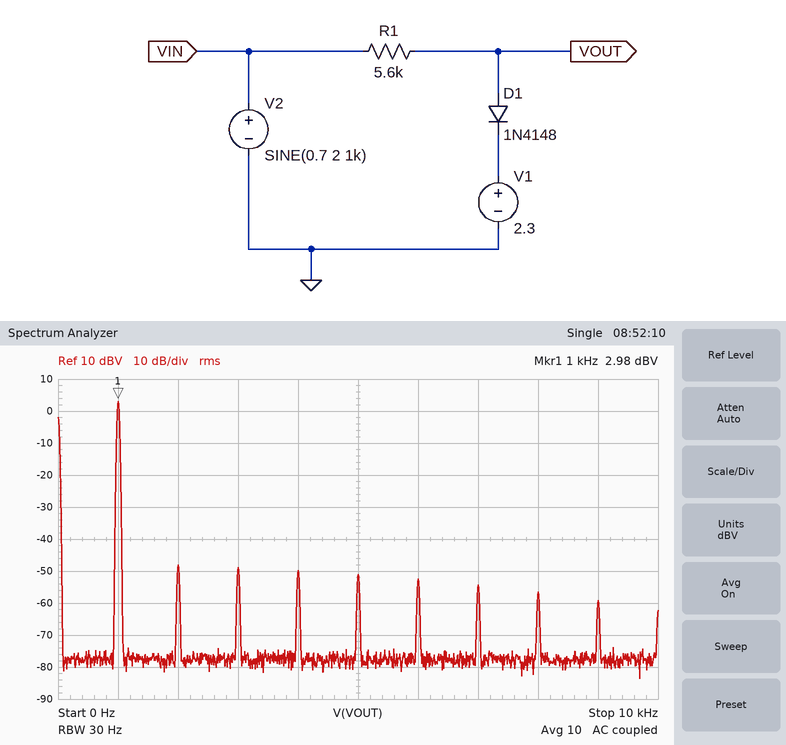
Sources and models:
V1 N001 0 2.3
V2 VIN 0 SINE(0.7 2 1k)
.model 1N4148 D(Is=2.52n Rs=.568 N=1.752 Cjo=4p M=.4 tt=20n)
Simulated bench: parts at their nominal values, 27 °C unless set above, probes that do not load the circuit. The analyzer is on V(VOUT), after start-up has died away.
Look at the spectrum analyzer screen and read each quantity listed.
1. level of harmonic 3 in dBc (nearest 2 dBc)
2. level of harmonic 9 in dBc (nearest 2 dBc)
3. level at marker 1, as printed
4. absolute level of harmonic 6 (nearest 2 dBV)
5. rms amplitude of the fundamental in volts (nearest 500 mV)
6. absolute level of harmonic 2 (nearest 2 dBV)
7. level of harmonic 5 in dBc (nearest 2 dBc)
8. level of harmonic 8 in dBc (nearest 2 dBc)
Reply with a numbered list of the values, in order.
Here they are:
1. -52 dBc
2. -62 dBc
3. 2.98 dBV
4. -52 dBV
5. 1.5 V
6. -48 dBV
7. -54 dBc
8. -60 dBc
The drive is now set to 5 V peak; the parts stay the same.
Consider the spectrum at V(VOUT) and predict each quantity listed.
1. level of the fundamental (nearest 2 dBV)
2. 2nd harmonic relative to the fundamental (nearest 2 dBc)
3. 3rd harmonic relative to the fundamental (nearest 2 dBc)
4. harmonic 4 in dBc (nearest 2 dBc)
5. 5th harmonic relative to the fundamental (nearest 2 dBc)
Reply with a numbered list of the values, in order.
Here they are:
1. 8 dBV
2. -14 dBc
3. -22 dBc
4. -56 dBc
5. -32 dBc
